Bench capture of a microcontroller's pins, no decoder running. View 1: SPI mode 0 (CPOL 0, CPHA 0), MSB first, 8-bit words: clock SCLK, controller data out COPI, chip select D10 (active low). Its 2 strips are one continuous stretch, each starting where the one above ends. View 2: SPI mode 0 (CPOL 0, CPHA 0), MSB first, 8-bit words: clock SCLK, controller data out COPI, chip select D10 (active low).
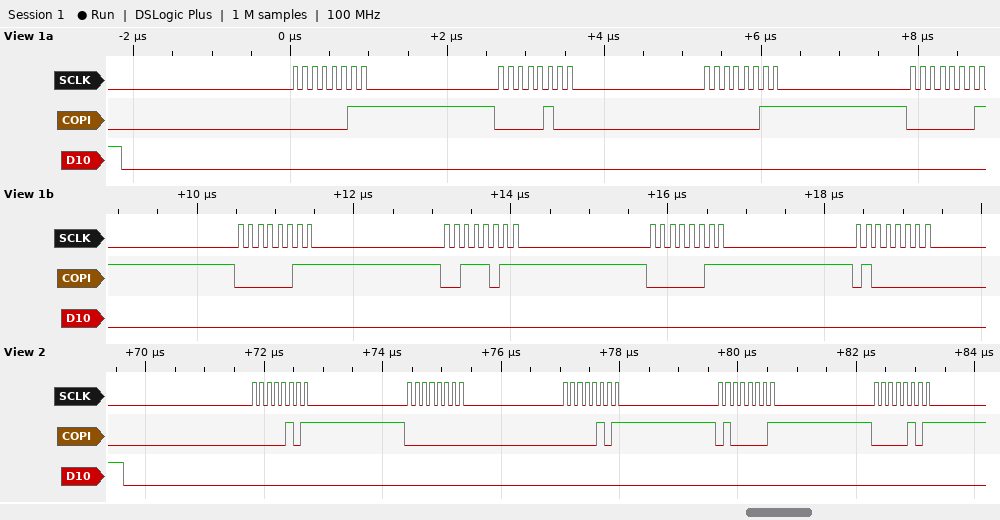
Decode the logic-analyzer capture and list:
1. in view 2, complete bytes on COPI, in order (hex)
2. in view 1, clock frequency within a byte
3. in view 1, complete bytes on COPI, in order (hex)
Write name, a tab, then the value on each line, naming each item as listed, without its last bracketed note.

in view 2, complete bytes on COPI, in order	05 00 05 41 05
in view 1, clock frequency within a byte	8 MHz
in view 1, complete bytes on COPI, in order	0x03 0x04 0x03 0x01 0x03 0x3B 0x03 0x40
